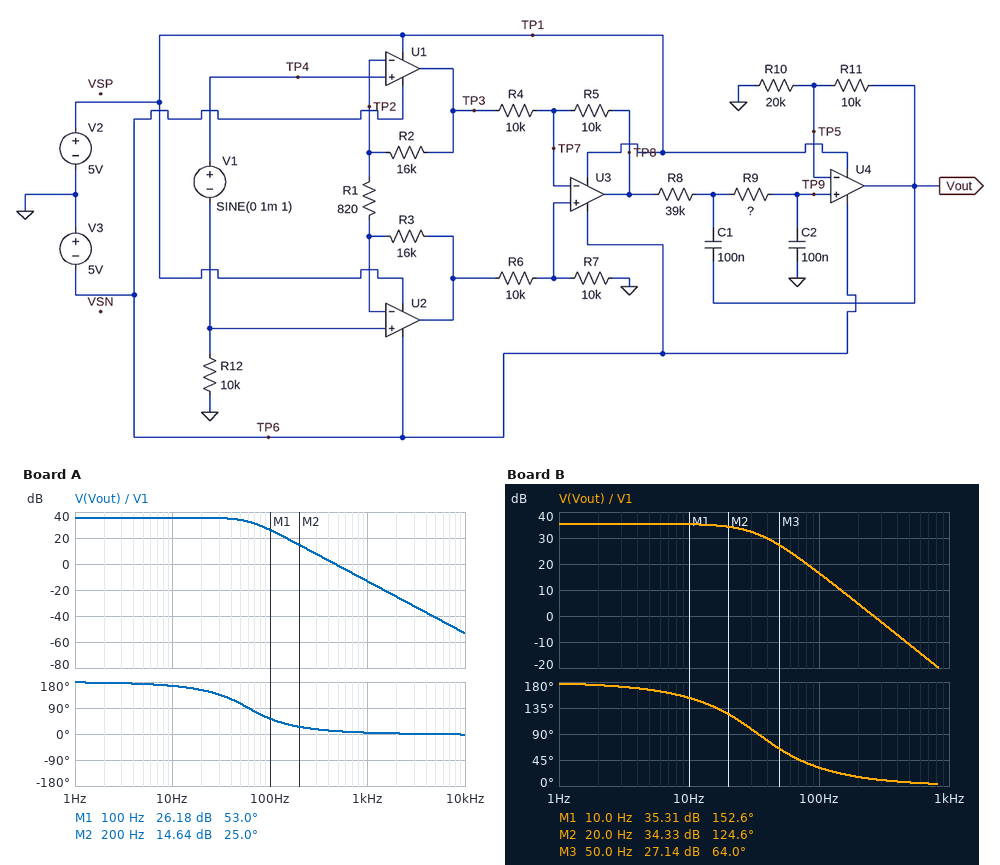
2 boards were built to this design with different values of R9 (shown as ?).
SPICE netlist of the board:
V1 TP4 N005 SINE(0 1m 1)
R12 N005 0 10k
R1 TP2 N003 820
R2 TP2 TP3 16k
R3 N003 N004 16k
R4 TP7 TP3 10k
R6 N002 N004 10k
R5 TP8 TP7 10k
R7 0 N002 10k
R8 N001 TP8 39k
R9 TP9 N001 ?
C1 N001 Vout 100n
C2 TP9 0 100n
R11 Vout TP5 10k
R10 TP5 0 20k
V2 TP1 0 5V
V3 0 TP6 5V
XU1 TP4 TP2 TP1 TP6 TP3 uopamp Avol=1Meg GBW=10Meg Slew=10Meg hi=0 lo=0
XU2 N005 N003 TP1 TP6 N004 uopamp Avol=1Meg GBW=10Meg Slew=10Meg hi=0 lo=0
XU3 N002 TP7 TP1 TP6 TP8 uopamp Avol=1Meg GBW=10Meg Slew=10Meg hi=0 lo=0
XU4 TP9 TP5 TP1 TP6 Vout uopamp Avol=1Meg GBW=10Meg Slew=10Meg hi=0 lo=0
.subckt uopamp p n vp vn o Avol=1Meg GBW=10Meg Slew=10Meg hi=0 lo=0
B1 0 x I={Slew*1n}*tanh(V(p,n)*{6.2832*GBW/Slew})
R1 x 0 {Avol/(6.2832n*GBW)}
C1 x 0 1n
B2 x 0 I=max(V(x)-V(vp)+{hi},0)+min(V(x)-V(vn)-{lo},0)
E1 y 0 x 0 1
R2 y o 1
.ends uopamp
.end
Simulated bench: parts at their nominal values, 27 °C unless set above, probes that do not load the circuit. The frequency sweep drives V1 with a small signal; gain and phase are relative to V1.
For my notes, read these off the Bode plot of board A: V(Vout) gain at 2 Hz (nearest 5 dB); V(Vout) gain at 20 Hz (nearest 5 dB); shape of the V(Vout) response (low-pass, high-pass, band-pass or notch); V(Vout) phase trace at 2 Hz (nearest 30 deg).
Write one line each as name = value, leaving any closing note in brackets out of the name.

V(Vout) gain at 2 Hz = 35 dB
V(Vout) gain at 20 Hz = 35 dB
shape of the V(Vout) response = low-pass
V(Vout) phase trace at 2 Hz = 180 deg
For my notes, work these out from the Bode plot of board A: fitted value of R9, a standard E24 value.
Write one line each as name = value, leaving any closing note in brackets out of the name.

fitted value of R9, a standard E24 value = 18 kΩ
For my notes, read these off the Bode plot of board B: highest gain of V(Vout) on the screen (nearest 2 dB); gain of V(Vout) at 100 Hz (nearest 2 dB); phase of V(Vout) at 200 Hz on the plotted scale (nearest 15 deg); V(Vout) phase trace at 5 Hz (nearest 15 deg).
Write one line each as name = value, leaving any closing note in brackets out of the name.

highest gain of V(Vout) on the screen = 36 dB
gain of V(Vout) at 100 Hz = 16 dB
phase of V(Vout) at 200 Hz on the plotted scale = 15 deg
V(Vout) phase trace at 5 Hz = 165 deg
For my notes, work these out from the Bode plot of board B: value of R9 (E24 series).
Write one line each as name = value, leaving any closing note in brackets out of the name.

value of R9 = 56 kΩ
